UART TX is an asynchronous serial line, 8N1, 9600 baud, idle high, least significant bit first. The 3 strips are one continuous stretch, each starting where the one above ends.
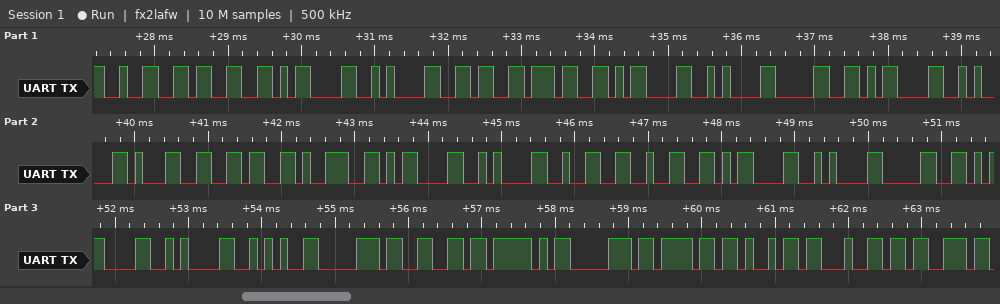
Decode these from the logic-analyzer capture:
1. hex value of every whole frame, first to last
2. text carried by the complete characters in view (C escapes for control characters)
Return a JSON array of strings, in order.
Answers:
["32 33 0D 0A 36 37 0D 0A 30 0D 0A 31 36 39 0D 0A 32 32 0D 0A 30 0D 0A 2A 70 66 5F 70 6F 69 64 73", "\"23\\r\\n67\\r\\n0\\r\\n169\\r\\n22\\r\\n0\\r\\n*pf_poids\""]
